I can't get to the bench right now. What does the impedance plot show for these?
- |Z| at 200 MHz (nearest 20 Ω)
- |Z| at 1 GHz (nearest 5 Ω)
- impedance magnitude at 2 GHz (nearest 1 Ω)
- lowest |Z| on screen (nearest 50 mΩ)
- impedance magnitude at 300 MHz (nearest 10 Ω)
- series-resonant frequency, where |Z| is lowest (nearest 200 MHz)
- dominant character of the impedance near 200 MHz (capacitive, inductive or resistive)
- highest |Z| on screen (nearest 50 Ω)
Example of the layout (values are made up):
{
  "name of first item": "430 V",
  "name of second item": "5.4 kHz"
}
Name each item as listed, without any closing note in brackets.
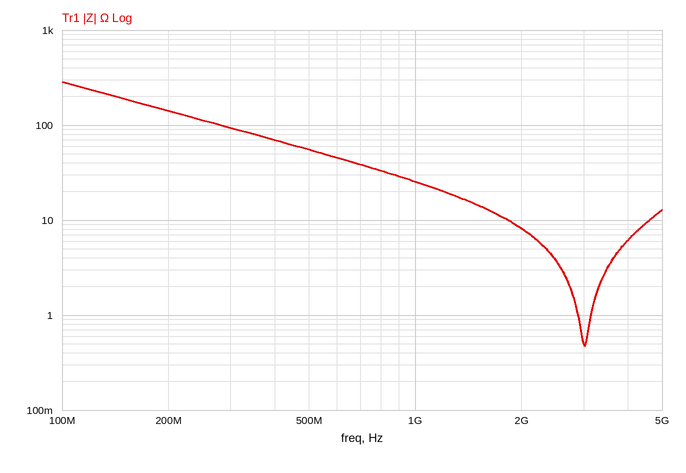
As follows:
{
  "|Z| at 200 MHz": "140 Ω",
  "|Z| at 1 GHz": "25 Ω",
  "impedance magnitude at 2 GHz": "8 Ω",
  "lowest |Z| on screen": "450 mΩ",
  "impedance magnitude at 300 MHz": "90 Ω",
  "series-resonant frequency, where |Z| is lowest": "3.0 GHz",
  "dominant character of the impedance near 200 MHz": "capacitive",
  "highest |Z| on screen": "300 Ω"
}
